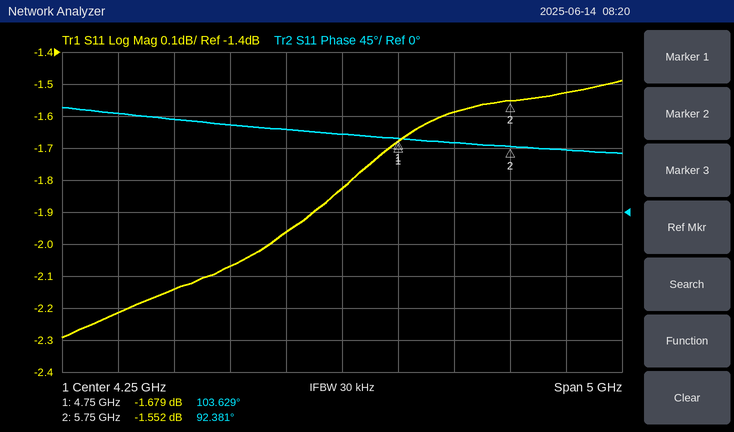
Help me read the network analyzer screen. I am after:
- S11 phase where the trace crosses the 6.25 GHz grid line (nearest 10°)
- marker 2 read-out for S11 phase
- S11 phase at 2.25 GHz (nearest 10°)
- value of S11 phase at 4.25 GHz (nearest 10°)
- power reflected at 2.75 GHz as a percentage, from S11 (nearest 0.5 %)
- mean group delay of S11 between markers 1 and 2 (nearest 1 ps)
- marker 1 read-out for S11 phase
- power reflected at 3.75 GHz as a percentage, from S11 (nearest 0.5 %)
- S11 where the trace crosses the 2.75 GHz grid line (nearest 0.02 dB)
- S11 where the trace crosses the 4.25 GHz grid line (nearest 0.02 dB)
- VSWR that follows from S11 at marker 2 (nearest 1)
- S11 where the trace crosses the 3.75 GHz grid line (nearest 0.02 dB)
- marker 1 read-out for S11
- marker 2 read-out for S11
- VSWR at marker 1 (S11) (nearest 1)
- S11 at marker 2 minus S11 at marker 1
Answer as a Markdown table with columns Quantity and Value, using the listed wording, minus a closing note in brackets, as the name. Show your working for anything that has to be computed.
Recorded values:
| Quantity | Value |
|---|---|
| S11 phase where the trace crosses the 6.25 GHz grid line | 90° |
| marker 2 read-out for S11 phase | 92.381° |
| S11 phase at 2.25 GHz | 140° |
| value of S11 phase at 4.25 GHz | 110° |
| power reflected at 2.75 GHz as a percentage, from S11 | 10^(-2.14/10) ≈ 61.1 %, so 61.0 % to the nearest 0.5 % |
| mean group delay of S11 between markers 1 and 2 | −(92.381° − (103.629°))/(360° × 1 GHz) ≈ 31 ps |
| marker 1 read-out for S11 phase | 103.629° |
| power reflected at 3.75 GHz as a percentage, from S11 | 10^(-1.96/10) ≈ 63.7 %, so 63.5 % to the nearest 0.5 % |
| S11 where the trace crosses the 2.75 GHz grid line | -2.14 dB |
| S11 where the trace crosses the 4.25 GHz grid line | -1.82 dB |
| VSWR that follows from S11 at marker 2 | (1 + 0.8364)/(1 − 0.8364) ≈ 11 |
| S11 where the trace crosses the 3.75 GHz grid line | -1.96 dB |
| marker 1 read-out for S11 | -1.679 dB |
| marker 2 read-out for S11 | -1.552 dB |
| VSWR at marker 1 (S11) | (1 + 0.8242)/(1 − 0.8242) ≈ 10 |
| S11 at marker 2 minus S11 at marker 1 | -1.552 − (-1.679) = 0.127 dB |
